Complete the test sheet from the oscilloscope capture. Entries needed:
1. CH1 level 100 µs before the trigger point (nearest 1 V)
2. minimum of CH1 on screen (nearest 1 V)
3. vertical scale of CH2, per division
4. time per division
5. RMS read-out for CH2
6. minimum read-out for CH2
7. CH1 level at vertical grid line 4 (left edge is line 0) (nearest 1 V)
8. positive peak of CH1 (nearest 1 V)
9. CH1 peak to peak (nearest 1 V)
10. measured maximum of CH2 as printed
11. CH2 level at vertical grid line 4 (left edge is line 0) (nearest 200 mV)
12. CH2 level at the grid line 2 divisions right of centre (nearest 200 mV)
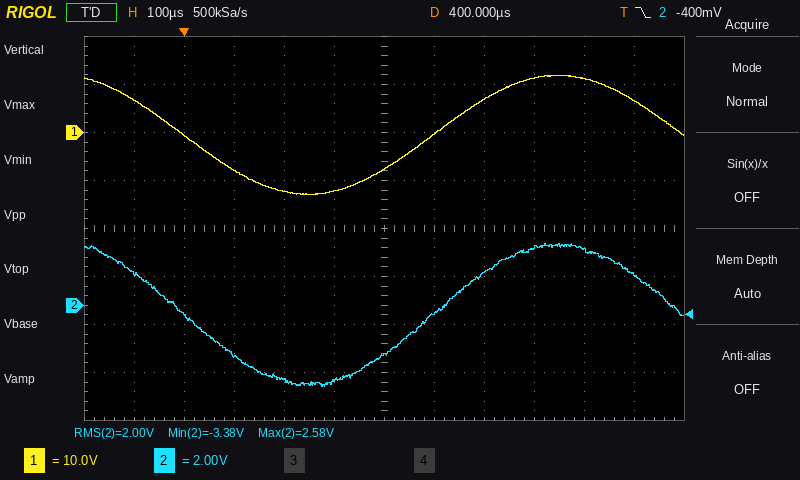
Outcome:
7 V
-13 V
2 V
100 µs
2.00 V
-3.38 V
-12 V
12 V
25 V
2.58 V
-3.2 V
1.4 V
